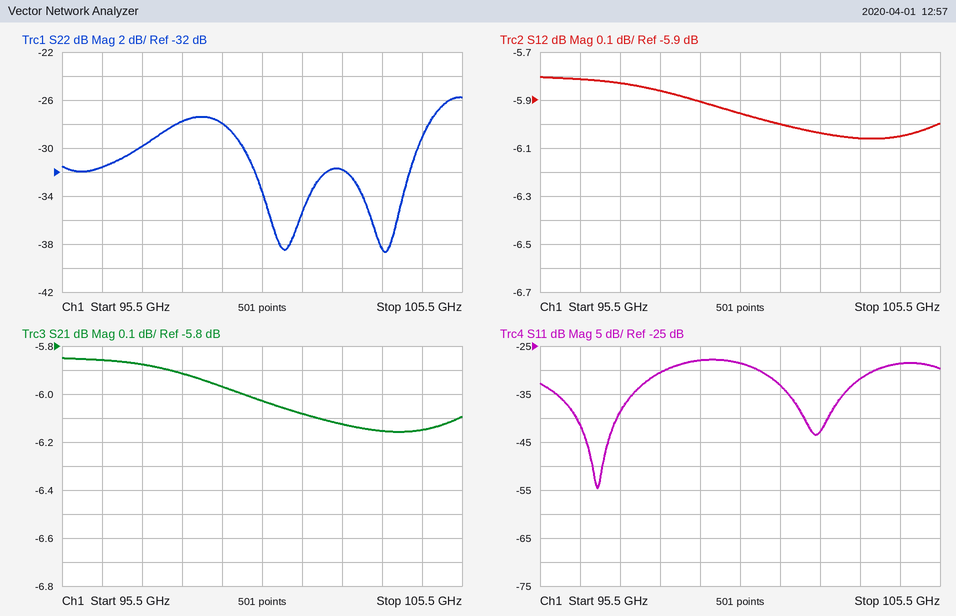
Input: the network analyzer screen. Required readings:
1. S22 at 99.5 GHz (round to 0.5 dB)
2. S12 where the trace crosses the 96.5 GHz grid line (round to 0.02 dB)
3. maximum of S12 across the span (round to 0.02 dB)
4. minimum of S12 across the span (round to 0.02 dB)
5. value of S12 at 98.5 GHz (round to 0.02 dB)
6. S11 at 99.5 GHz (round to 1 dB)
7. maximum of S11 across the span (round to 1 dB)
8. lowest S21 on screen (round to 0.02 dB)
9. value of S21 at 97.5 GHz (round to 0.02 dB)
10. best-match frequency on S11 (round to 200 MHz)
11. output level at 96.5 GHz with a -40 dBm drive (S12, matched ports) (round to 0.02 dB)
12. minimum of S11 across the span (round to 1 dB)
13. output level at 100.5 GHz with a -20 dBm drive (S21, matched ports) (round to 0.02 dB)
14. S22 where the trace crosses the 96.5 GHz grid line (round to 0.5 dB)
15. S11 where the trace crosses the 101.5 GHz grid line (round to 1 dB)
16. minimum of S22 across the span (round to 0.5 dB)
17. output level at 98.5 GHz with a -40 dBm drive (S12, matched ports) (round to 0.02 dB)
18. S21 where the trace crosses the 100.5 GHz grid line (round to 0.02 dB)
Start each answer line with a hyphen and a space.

- -28.0 dB
- -5.82 dB
- -5.80 dB
- -6.06 dB
- -5.86 dB
- -28 dB
- -28 dB
- -6.16 dB
- -5.88 dB
- 97.0 GHz
- -45.82 dBm
- -55 dB
- -26.02 dBm
- -31.5 dB
- -33 dB
- -38.5 dB
- -45.86 dBm
- -6.02 dB
